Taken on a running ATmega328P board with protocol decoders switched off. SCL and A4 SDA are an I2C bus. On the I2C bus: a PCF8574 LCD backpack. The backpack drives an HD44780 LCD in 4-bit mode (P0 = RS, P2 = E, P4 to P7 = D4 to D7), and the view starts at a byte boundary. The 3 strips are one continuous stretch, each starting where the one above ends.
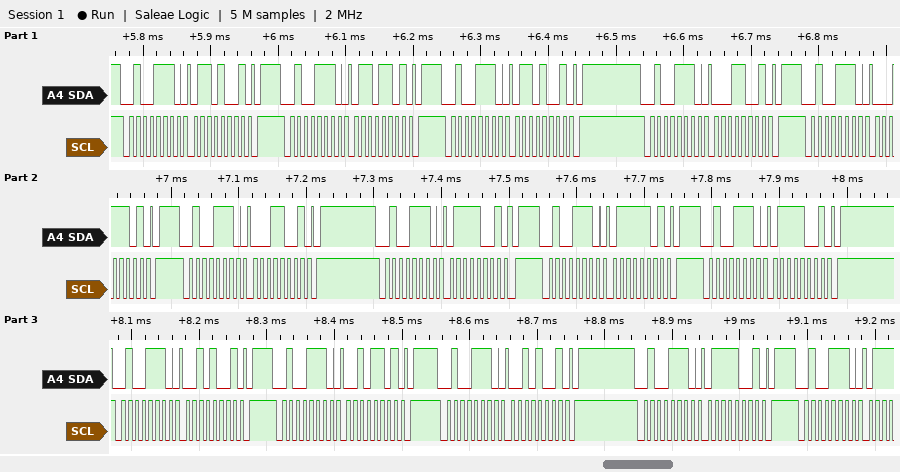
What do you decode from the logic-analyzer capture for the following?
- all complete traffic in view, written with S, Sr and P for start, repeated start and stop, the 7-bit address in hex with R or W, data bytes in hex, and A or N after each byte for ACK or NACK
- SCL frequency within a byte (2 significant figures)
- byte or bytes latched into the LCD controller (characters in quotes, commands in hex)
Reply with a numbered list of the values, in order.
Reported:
1. S 27W A 69 A P S 27W A 6D A P S 27W A 69 A P S 27W A 19 A P S 27W A 1D A P S 27W A 19 A P S 27W A 79 A P S 27W A 7D A P S 27W A 79 A P S 27W A 29 A P S 27W A 2D A P S 27W A 29 A P S 27W A 79 A P S 27W A
2. 100 kHz
3. 'a' 'r'
